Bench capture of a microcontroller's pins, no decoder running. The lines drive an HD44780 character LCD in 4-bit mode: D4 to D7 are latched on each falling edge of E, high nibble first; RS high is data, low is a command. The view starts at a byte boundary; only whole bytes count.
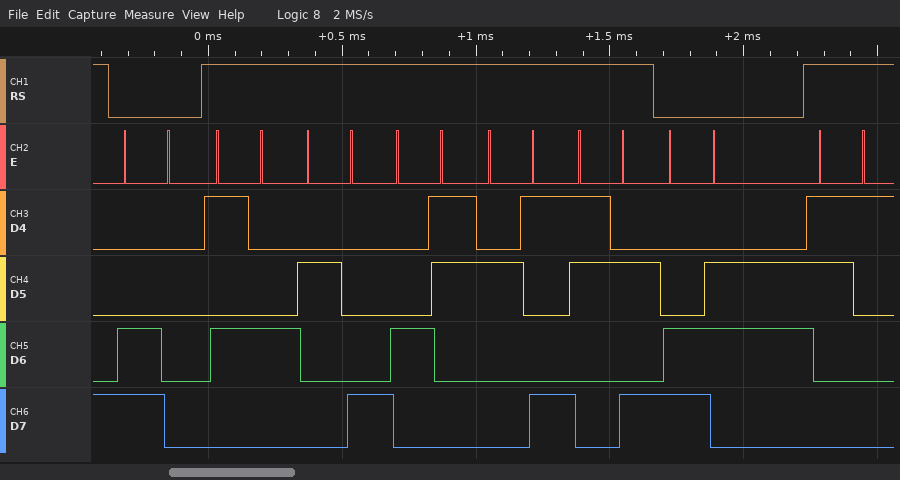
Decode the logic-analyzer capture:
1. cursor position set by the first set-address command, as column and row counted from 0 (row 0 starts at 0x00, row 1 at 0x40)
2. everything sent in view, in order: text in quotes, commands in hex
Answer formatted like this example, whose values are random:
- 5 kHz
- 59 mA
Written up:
- column 0, row 1
- 0xC0 "T(C):" 0xC6 "1"
